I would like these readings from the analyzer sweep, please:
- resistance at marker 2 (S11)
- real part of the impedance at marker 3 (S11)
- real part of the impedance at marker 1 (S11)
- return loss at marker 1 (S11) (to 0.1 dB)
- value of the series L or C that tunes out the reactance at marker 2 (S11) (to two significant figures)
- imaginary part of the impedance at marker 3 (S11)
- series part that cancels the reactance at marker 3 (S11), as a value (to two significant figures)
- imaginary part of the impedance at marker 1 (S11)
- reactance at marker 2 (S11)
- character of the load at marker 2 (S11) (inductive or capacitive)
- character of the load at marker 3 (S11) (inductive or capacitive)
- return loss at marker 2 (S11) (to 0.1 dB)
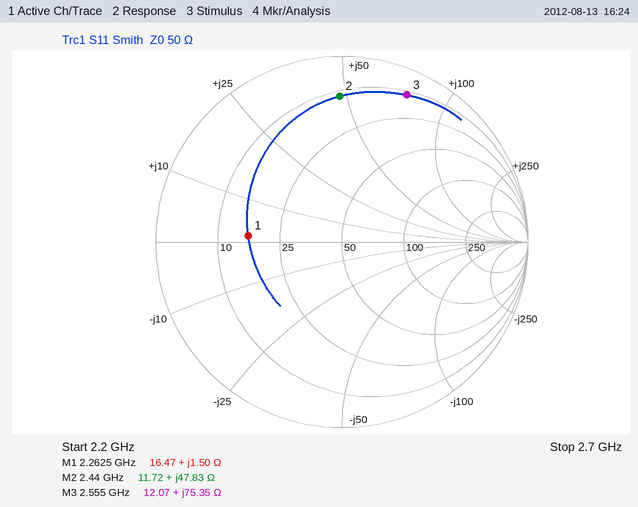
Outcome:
11.72 Ω
12.07 Ω
16.47 Ω
5.9 dB
1.4 pF
+75.35 Ω
830 fF
+1.50 Ω
+47.83 Ω
inductive
inductive
2.1 dB
